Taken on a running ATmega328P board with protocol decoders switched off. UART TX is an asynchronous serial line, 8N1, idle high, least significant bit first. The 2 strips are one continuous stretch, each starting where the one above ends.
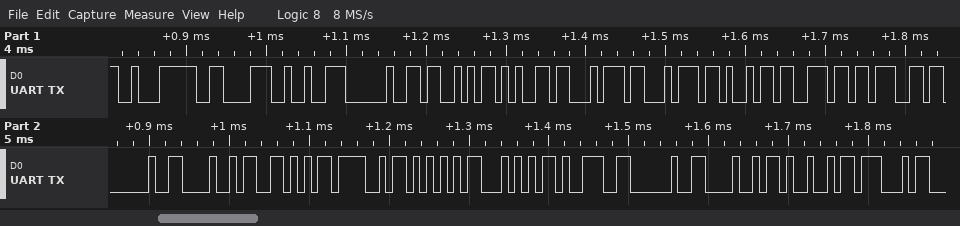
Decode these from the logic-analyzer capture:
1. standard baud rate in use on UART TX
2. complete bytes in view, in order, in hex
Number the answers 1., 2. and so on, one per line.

1. 115200 baud
2. E2 86 92 20 53 65 74 74 69 6E 67 20 48 56 4F 55 54 39 20 48 49 47
